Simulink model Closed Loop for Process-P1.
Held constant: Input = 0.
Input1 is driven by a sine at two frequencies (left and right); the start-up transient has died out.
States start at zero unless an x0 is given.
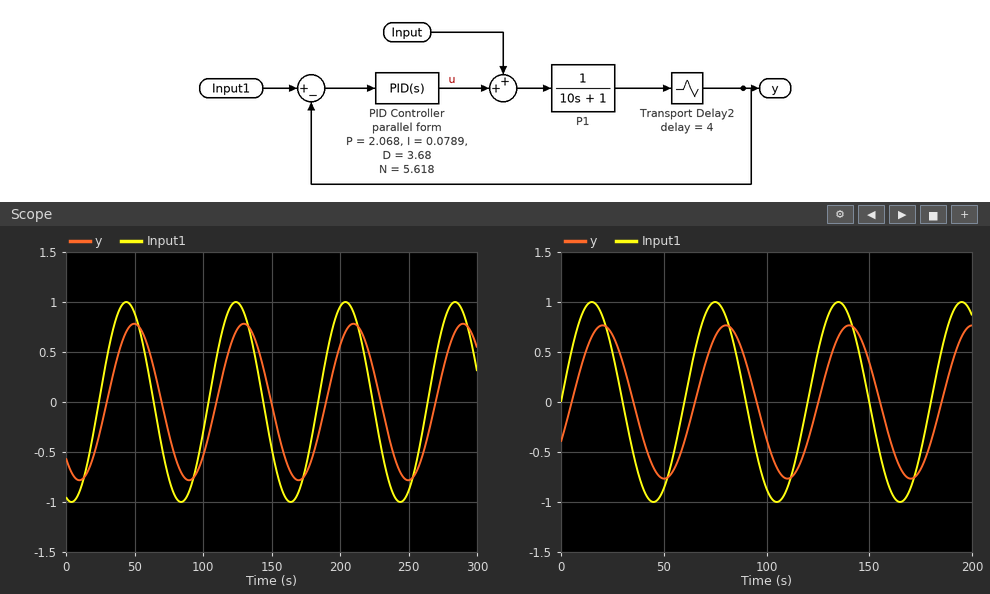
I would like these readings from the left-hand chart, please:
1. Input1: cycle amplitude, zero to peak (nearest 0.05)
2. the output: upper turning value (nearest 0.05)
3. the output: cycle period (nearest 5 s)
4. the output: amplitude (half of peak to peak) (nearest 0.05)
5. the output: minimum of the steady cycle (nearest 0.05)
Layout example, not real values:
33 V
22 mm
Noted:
1.00
0.80
80 s
0.80
-0.80
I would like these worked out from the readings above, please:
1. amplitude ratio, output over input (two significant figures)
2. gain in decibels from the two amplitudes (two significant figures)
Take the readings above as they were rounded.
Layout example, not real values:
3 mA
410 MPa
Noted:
0.80
-1.9 dB
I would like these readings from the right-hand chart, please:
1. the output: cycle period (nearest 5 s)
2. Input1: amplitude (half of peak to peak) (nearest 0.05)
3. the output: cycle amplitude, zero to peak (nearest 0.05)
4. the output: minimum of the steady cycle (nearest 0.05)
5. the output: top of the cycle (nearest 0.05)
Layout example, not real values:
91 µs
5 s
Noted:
60 s
1.00
0.75
-0.75
0.75
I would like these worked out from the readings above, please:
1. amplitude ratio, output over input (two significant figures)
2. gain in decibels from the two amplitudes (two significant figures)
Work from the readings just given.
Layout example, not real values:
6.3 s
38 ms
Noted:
0.75
-2.5 dB
